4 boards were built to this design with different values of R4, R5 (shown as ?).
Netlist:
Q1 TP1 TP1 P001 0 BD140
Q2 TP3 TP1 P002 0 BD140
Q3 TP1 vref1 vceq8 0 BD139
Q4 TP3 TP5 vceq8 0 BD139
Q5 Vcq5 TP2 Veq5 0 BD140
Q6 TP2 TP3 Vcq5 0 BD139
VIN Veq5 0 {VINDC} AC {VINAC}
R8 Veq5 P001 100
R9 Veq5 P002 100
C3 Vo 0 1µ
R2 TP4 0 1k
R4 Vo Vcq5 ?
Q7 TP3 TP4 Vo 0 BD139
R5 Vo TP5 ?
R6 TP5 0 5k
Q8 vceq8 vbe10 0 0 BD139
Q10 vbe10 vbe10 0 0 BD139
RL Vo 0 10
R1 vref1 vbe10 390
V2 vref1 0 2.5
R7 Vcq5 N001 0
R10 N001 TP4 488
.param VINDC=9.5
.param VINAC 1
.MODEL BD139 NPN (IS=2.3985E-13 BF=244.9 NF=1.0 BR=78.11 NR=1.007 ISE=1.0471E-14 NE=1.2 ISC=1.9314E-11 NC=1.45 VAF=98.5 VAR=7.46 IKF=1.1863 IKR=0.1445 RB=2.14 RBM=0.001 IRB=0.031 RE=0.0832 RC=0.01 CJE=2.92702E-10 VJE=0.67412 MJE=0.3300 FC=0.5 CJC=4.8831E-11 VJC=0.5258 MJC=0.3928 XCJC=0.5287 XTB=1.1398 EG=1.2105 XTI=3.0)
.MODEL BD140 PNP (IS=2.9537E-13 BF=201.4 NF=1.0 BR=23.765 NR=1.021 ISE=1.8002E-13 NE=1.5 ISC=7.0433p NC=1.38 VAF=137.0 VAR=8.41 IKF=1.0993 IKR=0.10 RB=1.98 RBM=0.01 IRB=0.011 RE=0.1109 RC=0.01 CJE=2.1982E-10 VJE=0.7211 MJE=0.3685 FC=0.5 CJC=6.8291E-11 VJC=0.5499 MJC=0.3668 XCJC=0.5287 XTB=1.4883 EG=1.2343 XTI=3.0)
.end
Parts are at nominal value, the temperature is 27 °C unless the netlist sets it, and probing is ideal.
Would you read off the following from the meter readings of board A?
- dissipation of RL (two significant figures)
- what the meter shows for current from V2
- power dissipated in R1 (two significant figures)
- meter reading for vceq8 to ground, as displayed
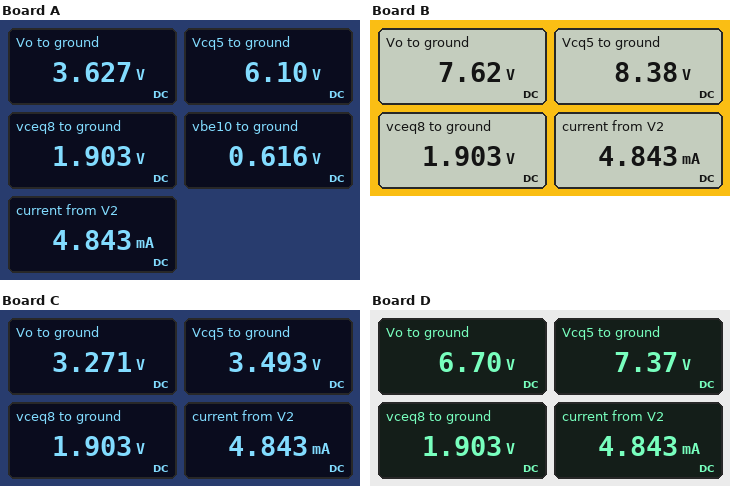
1.3 W
4.843 mA
9.1 mW
1.903 V
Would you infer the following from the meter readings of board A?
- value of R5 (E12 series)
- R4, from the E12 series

2.2 kΩ
6.8 Ω
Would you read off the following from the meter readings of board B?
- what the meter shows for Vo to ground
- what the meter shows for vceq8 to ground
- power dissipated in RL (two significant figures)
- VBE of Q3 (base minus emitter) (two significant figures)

7.62 V
1.903 V
5.8 W
600 mV
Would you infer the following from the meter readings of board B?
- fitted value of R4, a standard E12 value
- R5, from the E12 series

1 Ω
10 kΩ
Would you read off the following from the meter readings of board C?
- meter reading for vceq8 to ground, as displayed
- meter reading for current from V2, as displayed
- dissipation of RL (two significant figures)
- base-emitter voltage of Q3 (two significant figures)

1.903 V
4.843 mA
1.1 W
600 mV
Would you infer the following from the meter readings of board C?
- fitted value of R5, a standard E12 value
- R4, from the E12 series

1.5 kΩ
0.68 Ω
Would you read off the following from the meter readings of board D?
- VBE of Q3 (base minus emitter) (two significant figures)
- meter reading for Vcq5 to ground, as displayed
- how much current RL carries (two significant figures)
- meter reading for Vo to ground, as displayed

600 mV
7.37 V
670 mA
6.70 V
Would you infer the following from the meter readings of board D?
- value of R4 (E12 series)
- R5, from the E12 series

1 Ω
8.2 kΩ
